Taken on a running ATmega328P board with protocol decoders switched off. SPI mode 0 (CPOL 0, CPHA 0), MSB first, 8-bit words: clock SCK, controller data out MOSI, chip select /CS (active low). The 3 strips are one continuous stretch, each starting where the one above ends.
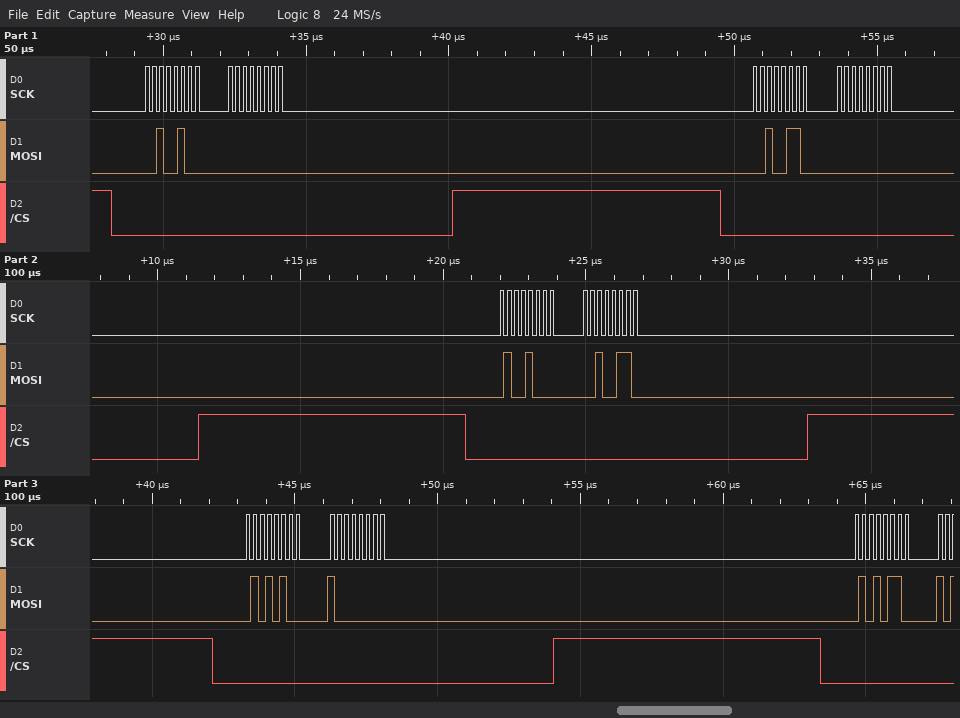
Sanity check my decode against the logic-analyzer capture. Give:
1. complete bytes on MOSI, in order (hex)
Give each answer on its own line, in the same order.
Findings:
0x24 0x00 0x26 0x00 0x48 0x26 0x54 0x80 0x56
